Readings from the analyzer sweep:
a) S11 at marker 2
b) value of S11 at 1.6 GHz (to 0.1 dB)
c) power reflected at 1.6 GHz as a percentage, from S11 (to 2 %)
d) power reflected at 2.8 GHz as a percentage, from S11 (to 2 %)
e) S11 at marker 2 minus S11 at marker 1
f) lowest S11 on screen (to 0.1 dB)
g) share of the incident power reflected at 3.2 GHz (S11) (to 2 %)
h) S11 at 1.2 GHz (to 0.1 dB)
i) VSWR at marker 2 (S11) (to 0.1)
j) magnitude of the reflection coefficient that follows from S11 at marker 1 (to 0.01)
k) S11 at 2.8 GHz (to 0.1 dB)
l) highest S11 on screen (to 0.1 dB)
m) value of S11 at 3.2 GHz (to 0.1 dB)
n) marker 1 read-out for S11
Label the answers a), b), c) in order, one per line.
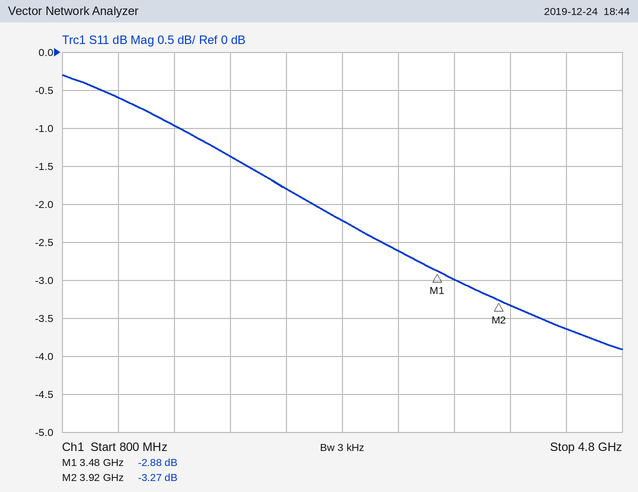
a) -3.27 dB
b) -1.0 dB
c) 80 %
d) 60 %
e) -0.39 dB
f) -3.9 dB
g) 54 %
h) -0.6 dB
i) 5.4
j) 0.72
k) -2.2 dB
l) -0.3 dB
m) -2.6 dB
n) -2.88 dB
